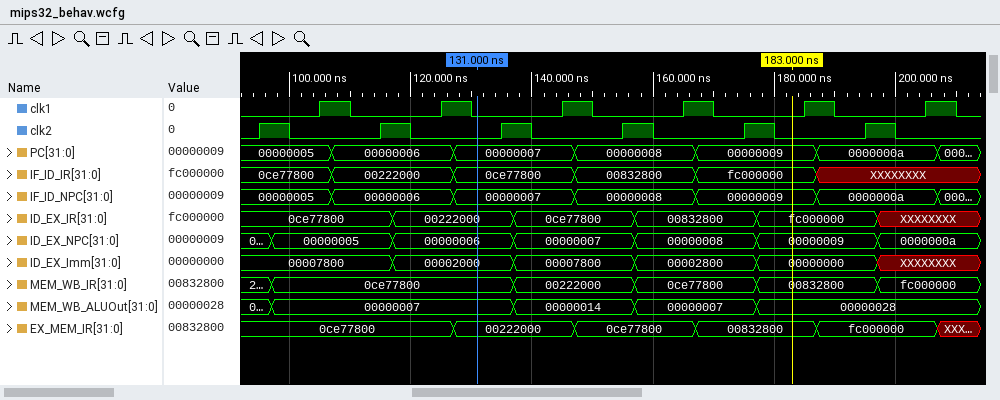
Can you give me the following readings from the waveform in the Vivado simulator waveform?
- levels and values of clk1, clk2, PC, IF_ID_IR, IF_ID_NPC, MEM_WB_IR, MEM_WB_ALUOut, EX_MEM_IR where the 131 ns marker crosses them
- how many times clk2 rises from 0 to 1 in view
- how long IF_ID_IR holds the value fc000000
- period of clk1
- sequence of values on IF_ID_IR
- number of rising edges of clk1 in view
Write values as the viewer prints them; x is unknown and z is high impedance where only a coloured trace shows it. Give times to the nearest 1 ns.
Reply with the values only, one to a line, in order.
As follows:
clk1=0, clk2=0, PC=00000007, IF_ID_IR=0ce77800, IF_ID_NPC=00000007, MEM_WB_IR=0ce77800, MEM_WB_ALUOut=00000007, EX_MEM_IR=00222000
6
20 ns
20 ns
0ce77800, 00222000, 0ce77800, 00832800, fc000000, XXXXXXXX
6
